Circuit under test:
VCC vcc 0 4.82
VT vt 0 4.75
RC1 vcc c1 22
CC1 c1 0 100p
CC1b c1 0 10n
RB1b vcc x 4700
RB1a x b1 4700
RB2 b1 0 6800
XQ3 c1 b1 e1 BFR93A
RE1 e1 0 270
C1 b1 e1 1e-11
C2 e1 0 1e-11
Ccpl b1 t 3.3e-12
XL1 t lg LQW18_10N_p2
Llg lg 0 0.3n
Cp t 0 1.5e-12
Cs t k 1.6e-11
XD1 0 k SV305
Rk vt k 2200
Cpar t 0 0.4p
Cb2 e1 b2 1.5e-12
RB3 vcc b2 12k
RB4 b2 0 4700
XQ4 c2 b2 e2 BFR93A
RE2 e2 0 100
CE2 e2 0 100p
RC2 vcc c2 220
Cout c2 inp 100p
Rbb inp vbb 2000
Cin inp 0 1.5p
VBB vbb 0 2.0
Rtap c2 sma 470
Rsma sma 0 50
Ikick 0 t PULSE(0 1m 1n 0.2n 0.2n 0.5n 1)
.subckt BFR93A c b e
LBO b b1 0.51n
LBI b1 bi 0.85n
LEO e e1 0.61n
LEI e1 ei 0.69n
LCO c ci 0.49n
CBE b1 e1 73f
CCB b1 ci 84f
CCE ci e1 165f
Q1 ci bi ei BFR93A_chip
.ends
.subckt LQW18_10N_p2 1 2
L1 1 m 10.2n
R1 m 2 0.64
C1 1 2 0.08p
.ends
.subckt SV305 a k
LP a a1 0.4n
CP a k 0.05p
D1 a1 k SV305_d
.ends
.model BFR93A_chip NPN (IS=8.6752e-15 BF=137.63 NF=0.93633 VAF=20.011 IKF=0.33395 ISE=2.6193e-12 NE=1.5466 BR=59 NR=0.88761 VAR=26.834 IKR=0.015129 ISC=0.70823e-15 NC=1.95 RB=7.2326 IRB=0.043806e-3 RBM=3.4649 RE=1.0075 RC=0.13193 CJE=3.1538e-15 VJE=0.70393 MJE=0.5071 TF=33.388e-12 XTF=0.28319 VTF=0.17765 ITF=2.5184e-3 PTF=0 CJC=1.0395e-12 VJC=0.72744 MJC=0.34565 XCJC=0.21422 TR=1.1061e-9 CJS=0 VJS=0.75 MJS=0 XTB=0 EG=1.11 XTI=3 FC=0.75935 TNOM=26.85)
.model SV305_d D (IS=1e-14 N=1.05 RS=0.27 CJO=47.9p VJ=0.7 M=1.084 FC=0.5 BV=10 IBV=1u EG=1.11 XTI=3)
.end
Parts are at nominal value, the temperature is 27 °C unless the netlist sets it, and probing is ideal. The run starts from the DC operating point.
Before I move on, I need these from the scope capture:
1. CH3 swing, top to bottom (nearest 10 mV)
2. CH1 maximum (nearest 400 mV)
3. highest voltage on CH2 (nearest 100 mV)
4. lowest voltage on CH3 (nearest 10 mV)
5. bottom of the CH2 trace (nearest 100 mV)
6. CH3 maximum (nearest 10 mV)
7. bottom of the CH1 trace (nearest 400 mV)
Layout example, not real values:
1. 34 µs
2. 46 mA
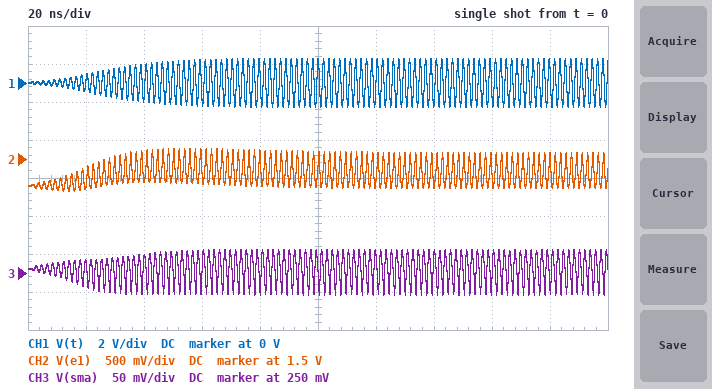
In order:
1. 60 mV
2. 1.2 V
3. 1.6 V
4. 220 mV
5. 1.1 V
6. 280 mV
7. -1.2 V
